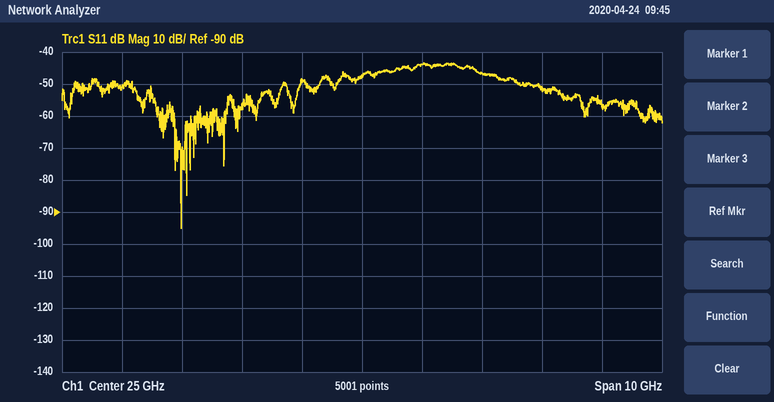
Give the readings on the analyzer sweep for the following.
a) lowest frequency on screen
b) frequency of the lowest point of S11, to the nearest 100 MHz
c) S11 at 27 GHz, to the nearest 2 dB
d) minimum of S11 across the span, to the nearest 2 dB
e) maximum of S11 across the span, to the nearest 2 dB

20 GHz
22.0 GHz
-46 dB
-96 dB
-44 dB
